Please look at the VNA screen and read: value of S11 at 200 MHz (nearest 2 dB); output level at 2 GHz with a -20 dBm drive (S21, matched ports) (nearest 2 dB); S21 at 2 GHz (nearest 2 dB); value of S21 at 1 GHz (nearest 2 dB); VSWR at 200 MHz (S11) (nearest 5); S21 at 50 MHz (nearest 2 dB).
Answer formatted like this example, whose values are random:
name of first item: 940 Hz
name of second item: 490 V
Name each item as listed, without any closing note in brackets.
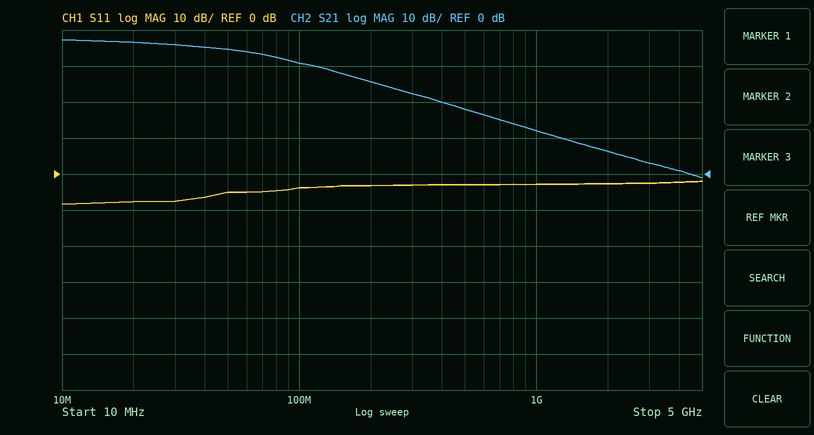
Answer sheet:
value of S11 at 200 MHz: -4 dB
output level at 2 GHz with a -20 dBm drive (S21, matched ports): -14 dBm
S21 at 2 GHz: 6 dB
value of S21 at 1 GHz: 12 dB
VSWR at 200 MHz (S11): 5
S21 at 50 MHz: 34 dB
